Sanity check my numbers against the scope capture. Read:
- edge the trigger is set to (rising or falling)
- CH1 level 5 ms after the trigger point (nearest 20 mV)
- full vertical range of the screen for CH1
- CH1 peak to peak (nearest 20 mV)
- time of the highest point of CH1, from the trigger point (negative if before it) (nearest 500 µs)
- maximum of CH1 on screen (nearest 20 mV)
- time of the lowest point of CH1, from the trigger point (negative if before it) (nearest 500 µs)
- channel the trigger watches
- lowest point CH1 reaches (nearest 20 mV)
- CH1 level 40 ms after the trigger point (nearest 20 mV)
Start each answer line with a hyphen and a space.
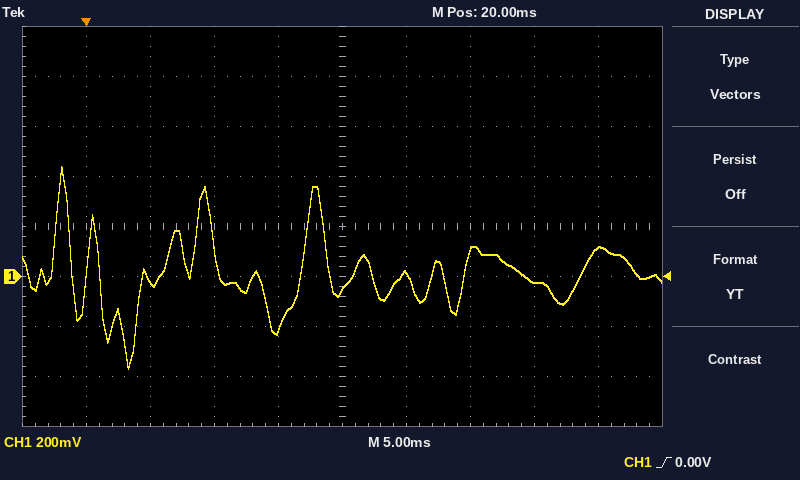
- rising
- -20 mV
- 1.6 V
- 800 mV
- -2.0 ms
- 440 mV
- +3.5 ms
- CH1
- -360 mV
- 120 mV
